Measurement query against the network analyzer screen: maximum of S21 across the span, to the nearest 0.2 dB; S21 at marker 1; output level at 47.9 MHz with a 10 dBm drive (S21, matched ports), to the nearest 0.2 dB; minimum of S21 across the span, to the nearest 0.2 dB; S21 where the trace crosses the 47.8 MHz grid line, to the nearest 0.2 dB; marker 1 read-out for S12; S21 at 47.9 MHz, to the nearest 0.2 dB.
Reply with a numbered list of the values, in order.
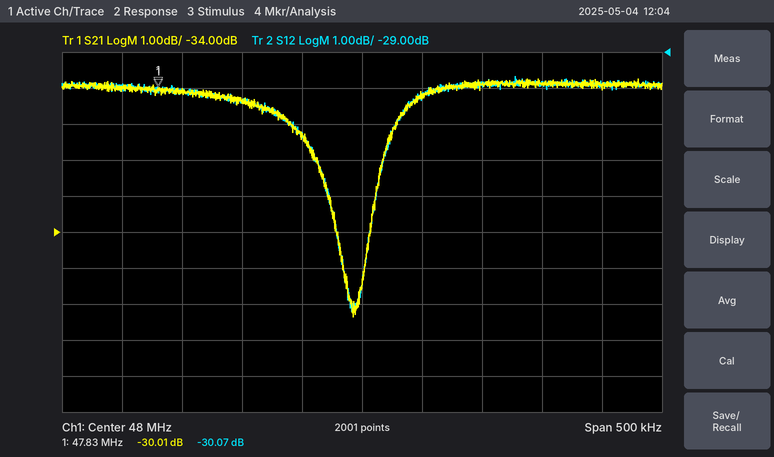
1. -29.8 dB
2. -30.01 dB
3. -20.4 dBm
4. -36.4 dB
5. -30.0 dB
6. -30.07 dB
7. -30.4 dB
